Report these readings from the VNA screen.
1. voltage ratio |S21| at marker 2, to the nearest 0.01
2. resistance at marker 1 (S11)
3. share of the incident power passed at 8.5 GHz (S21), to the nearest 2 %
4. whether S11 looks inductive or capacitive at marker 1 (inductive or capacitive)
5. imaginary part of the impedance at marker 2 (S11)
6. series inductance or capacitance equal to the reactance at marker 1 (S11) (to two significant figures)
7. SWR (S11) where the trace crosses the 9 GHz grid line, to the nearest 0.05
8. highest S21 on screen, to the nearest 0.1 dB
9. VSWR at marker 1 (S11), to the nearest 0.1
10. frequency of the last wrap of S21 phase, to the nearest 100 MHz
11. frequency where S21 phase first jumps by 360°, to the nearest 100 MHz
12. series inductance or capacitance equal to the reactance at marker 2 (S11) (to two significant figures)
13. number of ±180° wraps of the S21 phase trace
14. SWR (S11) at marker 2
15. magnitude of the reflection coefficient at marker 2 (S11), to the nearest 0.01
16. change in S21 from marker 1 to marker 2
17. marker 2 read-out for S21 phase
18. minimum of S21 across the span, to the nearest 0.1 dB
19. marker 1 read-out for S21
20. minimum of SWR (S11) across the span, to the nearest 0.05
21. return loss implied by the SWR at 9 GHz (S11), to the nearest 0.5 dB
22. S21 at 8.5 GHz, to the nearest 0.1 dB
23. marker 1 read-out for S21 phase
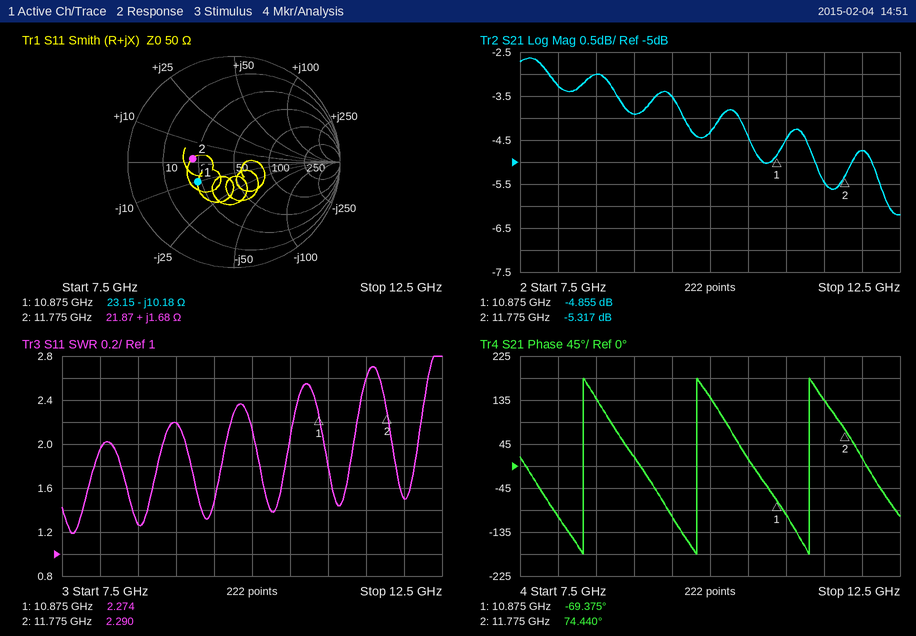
0.54
23.15 Ω
50 %
capacitive
+1.68 Ω
1.4 pF
2.20
-2.6 dB
2.3
11.3 GHz
8.3 GHz
23 pH
3
2.290
0.39
-0.462 dB
74.440°
-6.2 dB
-4.855 dB
1.20
8.5 dB
-3.0 dB
-69.375°
